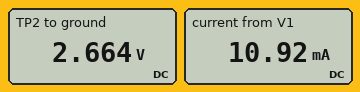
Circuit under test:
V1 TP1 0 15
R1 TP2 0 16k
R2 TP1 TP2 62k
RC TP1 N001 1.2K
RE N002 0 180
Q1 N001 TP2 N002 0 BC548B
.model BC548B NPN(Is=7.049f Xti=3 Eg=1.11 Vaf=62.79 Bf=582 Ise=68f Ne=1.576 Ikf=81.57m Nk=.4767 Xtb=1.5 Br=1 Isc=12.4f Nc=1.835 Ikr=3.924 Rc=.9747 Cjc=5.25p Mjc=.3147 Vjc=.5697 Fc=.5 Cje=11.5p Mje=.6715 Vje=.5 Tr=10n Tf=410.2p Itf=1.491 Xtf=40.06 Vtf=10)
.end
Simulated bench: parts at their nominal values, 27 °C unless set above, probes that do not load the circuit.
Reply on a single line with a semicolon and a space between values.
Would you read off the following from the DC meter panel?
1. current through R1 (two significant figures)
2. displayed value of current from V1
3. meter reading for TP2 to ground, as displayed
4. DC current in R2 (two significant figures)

170 µA; 10.92 mA; 2.664 V; 200 µA
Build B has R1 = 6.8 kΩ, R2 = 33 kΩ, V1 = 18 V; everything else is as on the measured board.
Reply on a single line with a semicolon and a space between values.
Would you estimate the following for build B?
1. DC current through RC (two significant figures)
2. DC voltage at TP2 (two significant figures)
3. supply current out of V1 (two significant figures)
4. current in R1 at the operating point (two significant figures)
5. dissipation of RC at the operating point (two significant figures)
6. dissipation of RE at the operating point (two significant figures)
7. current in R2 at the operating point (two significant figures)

12 mA; 2.9 V; 13 mA; 430 µA; 180 mW; 27 mW; 460 µA
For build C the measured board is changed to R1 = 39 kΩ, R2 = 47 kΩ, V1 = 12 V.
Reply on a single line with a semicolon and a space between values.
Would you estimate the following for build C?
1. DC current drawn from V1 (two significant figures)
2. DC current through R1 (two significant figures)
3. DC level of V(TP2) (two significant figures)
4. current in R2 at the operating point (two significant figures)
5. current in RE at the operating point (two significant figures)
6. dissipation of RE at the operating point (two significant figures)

8.8 mA; 59 µA; 2.3 V; 210 µA; 8.7 mA; 14 mW
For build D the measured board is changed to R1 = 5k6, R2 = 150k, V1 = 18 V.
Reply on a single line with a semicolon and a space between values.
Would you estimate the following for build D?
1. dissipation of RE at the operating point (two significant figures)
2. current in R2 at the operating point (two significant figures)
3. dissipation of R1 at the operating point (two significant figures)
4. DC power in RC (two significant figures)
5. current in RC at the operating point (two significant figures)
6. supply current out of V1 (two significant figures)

5.7 µW; 120 µA; 74 µW; 38 µW; 180 µA; 290 µA
